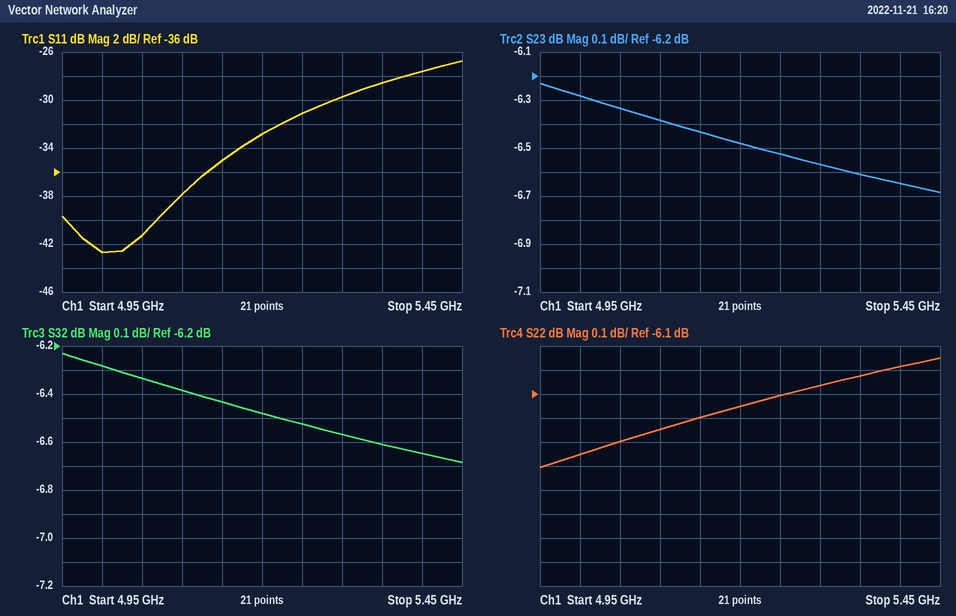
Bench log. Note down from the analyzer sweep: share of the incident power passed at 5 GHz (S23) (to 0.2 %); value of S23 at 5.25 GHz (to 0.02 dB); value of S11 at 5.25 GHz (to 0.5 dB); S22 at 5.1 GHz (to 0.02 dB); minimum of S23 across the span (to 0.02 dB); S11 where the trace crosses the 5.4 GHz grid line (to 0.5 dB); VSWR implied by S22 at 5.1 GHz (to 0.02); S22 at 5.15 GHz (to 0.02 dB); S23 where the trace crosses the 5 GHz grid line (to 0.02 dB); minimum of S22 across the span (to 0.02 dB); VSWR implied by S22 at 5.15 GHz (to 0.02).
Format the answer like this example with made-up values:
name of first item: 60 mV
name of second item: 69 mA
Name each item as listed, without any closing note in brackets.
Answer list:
share of the incident power passed at 5 GHz (S23): 23.6 %
value of S23 at 5.25 GHz: -6.52 dB
value of S11 at 5.25 GHz: -31.0 dB
S22 at 5.1 GHz: -6.24 dB
minimum of S23 across the span: -6.68 dB
S11 where the trace crosses the 5.4 GHz grid line: -27.5 dB
VSWR implied by S22 at 5.1 GHz: 2.90
S22 at 5.15 GHz: -6.20 dB
S23 where the trace crosses the 5 GHz grid line: -6.28 dB
minimum of S22 across the span: -6.40 dB
VSWR implied by S22 at 5.15 GHz: 2.92
